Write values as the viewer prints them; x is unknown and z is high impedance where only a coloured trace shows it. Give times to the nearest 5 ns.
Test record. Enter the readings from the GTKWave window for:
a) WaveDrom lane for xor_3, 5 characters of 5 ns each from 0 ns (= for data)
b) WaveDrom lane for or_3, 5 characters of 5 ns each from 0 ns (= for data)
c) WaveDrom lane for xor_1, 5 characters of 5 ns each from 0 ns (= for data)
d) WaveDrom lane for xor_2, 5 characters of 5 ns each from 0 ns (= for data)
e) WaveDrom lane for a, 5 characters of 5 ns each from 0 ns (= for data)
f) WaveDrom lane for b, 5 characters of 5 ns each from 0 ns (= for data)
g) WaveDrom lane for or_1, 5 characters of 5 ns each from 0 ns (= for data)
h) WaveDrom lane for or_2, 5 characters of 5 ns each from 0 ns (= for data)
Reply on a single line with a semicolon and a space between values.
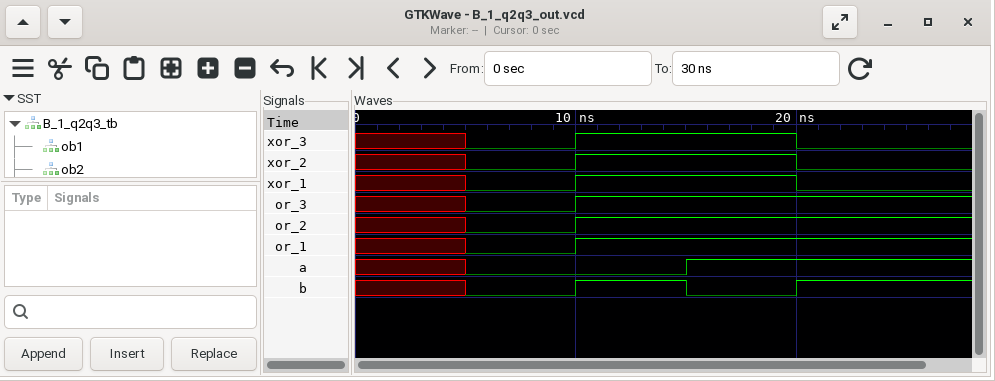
{name: 'xor_3', wave: 'x01.0'}; {name: 'or_3', wave: 'x01..'}; {name: 'xor_1', wave: 'x01.0'}; {name: 'xor_2', wave: 'x01.0'}; {name: 'a', wave: 'x0.1.'}; {name: 'b', wave: 'x0101'}; {name: 'or_1', wave: 'x01..'}; {name: 'or_2', wave: 'x01..'}
